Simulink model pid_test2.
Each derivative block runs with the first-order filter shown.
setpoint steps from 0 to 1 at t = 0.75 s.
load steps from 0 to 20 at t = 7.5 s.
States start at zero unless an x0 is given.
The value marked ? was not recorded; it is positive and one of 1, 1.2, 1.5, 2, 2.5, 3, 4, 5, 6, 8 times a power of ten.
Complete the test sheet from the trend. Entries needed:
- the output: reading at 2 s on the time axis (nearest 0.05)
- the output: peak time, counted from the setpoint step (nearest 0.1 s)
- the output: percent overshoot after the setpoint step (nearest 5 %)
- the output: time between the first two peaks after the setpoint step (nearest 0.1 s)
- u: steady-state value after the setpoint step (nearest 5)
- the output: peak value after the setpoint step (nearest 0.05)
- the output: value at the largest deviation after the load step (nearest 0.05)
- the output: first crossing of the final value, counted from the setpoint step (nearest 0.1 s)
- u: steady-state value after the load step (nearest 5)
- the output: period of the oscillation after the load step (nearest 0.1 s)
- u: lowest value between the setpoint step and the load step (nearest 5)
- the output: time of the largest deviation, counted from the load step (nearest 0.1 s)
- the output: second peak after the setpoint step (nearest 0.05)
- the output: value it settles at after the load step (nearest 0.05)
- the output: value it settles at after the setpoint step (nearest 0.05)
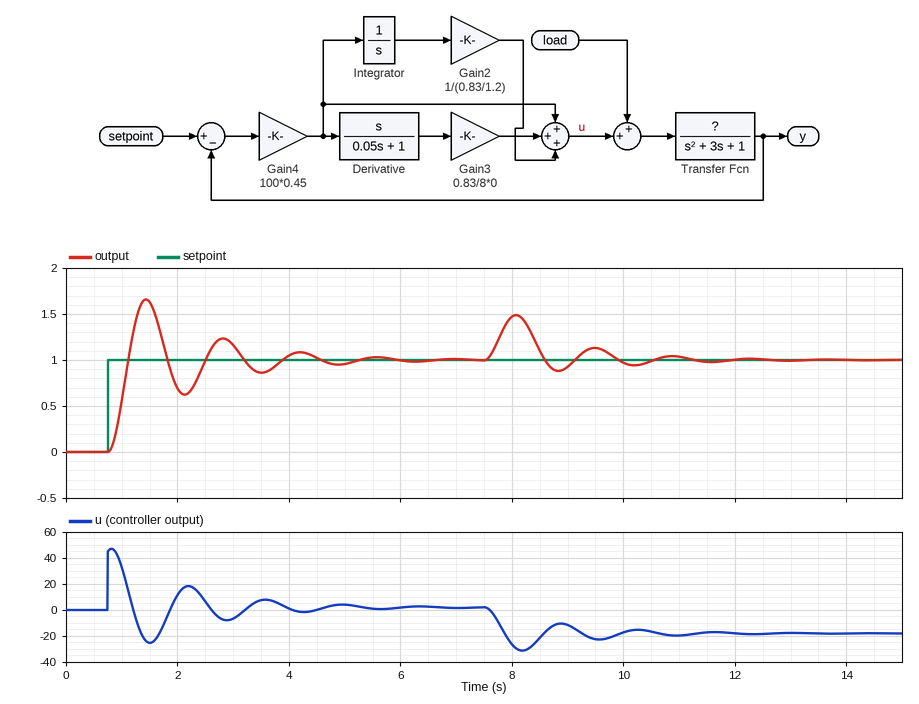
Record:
0.70
0.7 s
65 %
1.4 s
0
1.65
1.50
0.4 s
-20
1.4 s
-25
0.6 s
1.25
1.00
1.00
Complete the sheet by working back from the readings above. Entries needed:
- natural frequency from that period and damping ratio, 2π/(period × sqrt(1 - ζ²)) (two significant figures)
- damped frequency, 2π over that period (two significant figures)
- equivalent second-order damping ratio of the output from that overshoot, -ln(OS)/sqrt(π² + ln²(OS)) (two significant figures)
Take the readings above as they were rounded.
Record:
4.5 rad/s
4.5 rad/s
0.14
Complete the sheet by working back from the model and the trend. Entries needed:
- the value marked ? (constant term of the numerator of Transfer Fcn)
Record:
0.5
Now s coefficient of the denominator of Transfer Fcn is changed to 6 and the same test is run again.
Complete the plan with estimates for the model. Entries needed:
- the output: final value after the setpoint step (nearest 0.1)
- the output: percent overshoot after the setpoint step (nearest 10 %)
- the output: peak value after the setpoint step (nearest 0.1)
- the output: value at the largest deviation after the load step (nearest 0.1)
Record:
1.0
40 %
1.4
1.4
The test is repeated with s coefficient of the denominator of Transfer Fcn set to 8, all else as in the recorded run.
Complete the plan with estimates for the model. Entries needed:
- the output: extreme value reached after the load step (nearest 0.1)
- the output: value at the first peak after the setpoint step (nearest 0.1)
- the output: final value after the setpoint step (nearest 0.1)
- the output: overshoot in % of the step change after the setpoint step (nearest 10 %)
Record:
1.3
1.3
1.0
30 %
